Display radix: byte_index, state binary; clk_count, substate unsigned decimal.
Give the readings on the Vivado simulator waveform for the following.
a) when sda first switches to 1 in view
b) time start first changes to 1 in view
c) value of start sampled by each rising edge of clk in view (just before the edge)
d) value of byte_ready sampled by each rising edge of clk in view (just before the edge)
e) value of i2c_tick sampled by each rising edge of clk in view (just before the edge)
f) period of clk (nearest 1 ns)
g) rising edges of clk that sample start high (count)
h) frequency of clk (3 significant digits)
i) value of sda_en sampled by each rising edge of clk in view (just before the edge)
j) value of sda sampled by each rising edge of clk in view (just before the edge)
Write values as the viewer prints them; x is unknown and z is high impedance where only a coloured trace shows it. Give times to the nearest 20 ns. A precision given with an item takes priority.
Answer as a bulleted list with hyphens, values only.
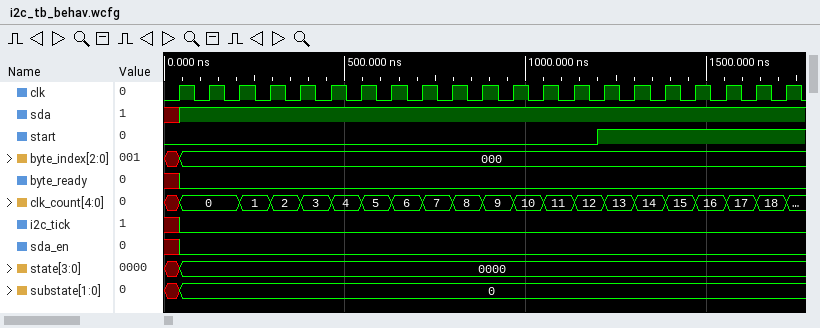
- 40 ns
- 1200 ns
- 0 0 0 0 0 0 0 0 0 0 0 0 0 0 1 1 1 1 1 1 1
- x 0 0 0 0 0 0 0 0 0 0 0 0 0 0 0 0 0 0 0 0
- x 0 0 0 0 0 0 0 0 0 0 0 0 0 0 0 0 0 0 0 0
- 84 ns
- 7
- 11.9 MHz
- x 0 0 0 0 0 0 0 0 0 0 0 0 0 0 0 0 0 0 0 0
- x 1 1 1 1 1 1 1 1 1 1 1 1 1 1 1 1 1 1 1 1
